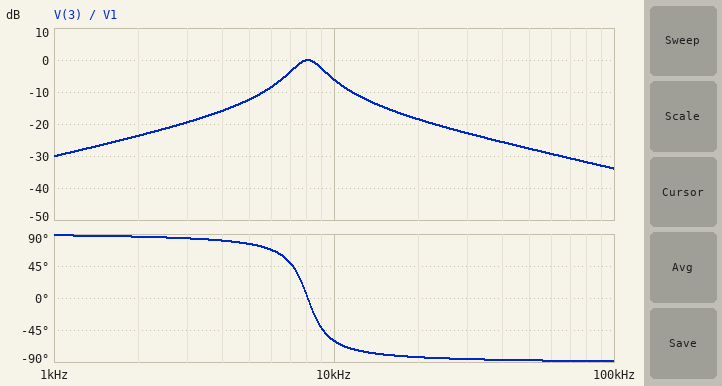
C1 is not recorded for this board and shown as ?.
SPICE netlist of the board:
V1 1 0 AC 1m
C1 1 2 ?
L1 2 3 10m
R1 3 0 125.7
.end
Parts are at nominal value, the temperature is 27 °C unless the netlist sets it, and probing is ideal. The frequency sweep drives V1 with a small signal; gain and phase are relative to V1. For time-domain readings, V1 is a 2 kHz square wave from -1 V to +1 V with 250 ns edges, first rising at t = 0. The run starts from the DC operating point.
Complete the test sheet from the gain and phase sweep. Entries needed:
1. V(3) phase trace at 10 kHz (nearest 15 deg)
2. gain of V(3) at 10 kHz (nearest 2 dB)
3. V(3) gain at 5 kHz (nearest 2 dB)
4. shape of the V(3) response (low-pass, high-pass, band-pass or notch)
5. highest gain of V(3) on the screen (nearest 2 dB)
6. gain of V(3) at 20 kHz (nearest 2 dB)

-60 deg
-6 dB
-12 dB
band-pass
0 dB
-18 dB
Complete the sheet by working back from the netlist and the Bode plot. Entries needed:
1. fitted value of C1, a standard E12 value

39 nF
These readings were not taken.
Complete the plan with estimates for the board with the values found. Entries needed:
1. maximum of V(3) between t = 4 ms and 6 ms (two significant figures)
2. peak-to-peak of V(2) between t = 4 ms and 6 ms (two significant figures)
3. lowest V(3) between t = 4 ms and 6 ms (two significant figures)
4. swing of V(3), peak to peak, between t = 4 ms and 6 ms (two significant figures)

340 mV
3.3 V
-340 mV
690 mV
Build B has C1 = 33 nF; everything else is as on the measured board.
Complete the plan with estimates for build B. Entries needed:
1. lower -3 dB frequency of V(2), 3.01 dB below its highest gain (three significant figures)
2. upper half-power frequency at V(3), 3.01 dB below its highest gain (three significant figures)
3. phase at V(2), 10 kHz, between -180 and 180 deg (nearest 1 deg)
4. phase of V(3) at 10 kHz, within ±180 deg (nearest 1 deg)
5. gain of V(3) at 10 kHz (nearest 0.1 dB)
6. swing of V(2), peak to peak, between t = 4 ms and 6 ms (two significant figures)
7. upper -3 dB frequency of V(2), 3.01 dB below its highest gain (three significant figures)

7.99 kHz
9.82 kHz
29 deg
-49 deg
-3.7 dB
3.5 V
10.1 kHz
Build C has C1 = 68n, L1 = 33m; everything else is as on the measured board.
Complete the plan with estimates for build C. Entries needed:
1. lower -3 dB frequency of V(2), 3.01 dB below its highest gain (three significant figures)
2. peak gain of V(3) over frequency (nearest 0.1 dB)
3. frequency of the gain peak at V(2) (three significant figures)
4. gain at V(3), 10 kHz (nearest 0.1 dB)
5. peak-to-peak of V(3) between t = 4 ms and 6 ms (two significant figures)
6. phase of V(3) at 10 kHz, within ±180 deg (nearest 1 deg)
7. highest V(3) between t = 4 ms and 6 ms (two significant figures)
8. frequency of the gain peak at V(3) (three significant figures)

3.11 kHz
0 dB
3.39 kHz
-23.3 dB
460 mV
-86 deg
230 mV
3.36 kHz
